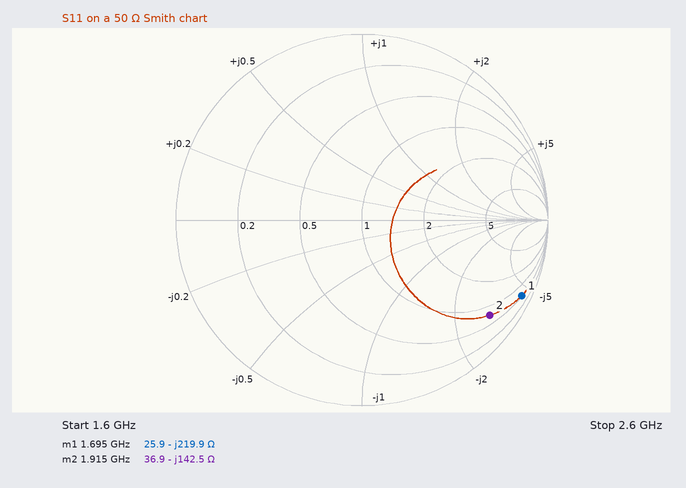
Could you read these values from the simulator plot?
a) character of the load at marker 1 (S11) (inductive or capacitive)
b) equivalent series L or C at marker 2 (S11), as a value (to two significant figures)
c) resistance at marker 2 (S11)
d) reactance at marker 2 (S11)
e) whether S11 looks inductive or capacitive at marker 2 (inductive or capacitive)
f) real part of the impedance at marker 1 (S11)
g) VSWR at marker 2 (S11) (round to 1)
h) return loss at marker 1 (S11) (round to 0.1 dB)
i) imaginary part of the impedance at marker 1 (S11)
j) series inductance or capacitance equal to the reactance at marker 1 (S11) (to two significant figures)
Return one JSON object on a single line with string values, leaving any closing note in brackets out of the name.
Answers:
{"character of the load at marker 1 (S11)": "capacitive", "equivalent series L or C at marker 2 (S11), as a value": "580 fF", "resistance at marker 2": "36.9 Ω", "reactance at marker 2": "-142.5 Ω", "whether S11 looks inductive or capacitive at marker 2": "capacitive", "real part of the impedance at marker 1": "25.9 Ω", "VSWR at marker 2 (S11)": "13", "return loss at marker 1 (S11)": "0.4 dB", "imaginary part of the impedance at marker 1": "-219.9 Ω", "series inductance or capacitance equal to the reactance at marker 1 (S11)": "430 fF"}
